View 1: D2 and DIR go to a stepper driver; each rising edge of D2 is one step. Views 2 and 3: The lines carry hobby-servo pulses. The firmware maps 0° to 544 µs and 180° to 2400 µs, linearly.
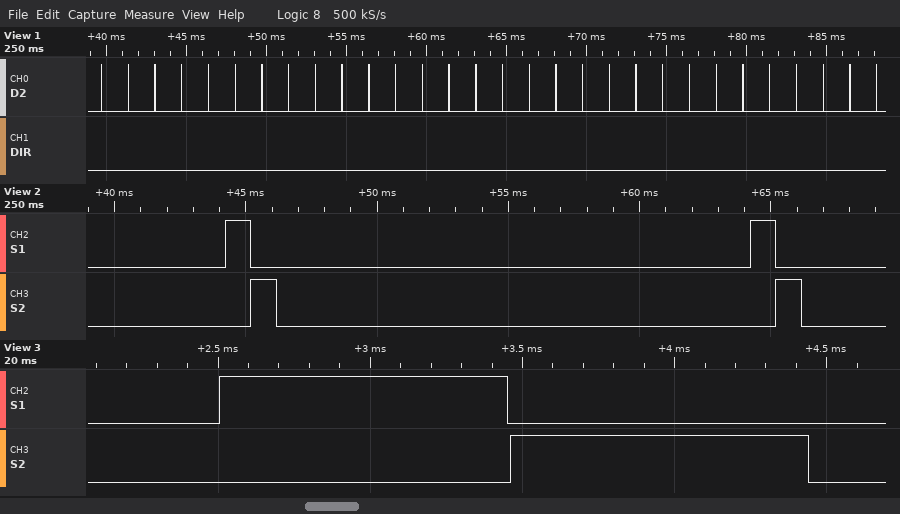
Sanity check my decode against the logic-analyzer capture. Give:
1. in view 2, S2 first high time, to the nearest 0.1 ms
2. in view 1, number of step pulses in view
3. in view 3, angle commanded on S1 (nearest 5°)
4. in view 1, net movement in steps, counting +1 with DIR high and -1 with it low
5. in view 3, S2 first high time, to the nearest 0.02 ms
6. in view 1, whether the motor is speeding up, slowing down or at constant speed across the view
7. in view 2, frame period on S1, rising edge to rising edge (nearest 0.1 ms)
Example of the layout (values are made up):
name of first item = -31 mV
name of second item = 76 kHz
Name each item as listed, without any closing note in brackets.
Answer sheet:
in view 2, S2 first high time, to the nearest 0.1 ms = 1.0 ms
in view 1, number of step pulses in view = 30
in view 3, angle commanded on S1 = 40°
in view 1, net movement in steps, counting +1 with DIR high and -1 with it low = -30
in view 3, S2 first high time, to the nearest 0.02 ms = 0.98 ms
in view 1, whether the motor is speeding up, slowing down or at constant speed across the view = constant speed
in view 2, frame period on S1, rising edge to rising edge = 20.0 ms
